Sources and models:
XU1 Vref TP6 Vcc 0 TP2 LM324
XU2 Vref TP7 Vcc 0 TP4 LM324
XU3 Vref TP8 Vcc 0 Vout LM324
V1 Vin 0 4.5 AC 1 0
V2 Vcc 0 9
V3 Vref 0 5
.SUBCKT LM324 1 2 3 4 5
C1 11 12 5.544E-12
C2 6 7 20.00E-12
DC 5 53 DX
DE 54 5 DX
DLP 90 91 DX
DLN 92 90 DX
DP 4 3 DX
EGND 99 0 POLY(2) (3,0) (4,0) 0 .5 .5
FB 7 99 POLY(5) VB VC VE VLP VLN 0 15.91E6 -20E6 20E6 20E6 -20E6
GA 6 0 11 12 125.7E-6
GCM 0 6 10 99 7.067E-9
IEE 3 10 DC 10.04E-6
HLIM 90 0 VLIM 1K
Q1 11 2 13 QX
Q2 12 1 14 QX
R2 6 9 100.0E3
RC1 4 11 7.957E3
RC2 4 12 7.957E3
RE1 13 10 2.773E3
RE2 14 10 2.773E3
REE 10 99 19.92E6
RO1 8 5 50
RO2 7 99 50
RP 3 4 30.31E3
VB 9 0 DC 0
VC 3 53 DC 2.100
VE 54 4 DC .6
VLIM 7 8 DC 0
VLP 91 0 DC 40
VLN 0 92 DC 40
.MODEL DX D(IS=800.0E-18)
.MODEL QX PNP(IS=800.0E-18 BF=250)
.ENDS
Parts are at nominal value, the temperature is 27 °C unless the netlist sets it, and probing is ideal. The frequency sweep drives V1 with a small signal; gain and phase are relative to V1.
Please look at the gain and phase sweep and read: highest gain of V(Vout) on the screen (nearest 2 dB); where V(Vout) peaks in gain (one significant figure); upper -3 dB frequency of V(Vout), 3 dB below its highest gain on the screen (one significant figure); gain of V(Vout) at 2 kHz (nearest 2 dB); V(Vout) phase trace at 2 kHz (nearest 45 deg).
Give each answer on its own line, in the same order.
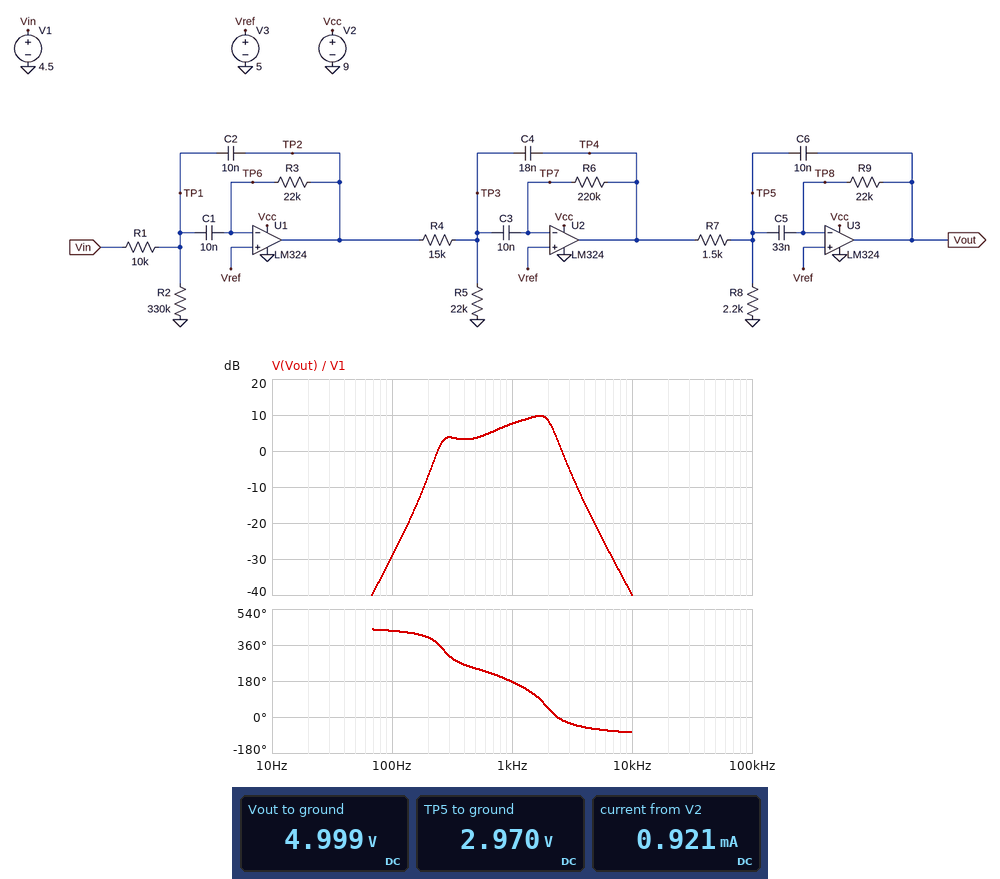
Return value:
10 dB
2 kHz
2 kHz
8 dB
45 deg
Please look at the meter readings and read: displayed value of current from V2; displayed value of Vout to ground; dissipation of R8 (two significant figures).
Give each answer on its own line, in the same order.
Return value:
0.921 mA
4.999 V
4.0 mW
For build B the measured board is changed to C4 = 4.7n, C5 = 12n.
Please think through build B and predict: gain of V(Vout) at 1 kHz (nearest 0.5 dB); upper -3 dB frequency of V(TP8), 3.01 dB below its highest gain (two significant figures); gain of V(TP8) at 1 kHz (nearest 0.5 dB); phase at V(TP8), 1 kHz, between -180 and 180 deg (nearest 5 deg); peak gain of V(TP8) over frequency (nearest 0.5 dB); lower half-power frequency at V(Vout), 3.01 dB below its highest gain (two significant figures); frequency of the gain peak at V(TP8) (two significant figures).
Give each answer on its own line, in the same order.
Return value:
11.0 dB
3.7 kHz
-49.0 dB
105 deg
-40.5 dB
480 Hz
3.1 kHz
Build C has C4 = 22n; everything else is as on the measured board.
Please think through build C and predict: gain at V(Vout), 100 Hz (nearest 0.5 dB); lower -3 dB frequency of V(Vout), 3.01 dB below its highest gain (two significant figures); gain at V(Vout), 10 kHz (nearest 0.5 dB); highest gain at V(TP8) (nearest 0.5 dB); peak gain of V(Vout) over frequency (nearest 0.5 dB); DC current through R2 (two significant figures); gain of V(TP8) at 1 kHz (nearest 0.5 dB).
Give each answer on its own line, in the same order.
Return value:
-29.0 dB
880 Hz
-41.5 dB
-47.0 dB
8.0 dB
13 µA
-54.0 dB
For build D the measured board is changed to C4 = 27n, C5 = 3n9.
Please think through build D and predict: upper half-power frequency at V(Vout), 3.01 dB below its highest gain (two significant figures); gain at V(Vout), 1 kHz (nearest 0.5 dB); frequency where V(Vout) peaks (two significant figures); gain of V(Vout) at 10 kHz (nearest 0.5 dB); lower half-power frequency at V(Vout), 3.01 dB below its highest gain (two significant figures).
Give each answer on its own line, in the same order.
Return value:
2.2 kHz
-16.5 dB
1.1 kHz
-41.0 dB
520 Hz
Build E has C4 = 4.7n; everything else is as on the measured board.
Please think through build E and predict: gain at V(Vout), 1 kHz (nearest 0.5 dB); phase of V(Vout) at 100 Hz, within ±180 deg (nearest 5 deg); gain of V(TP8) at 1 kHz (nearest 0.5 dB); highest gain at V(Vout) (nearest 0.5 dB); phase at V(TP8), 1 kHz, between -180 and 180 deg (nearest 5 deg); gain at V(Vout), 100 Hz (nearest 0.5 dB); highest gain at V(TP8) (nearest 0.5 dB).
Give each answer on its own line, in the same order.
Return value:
21.0 dB
75 deg
-39.0 dB
22.0 dB
95 deg
-30.0 dB
-33.0 dB
